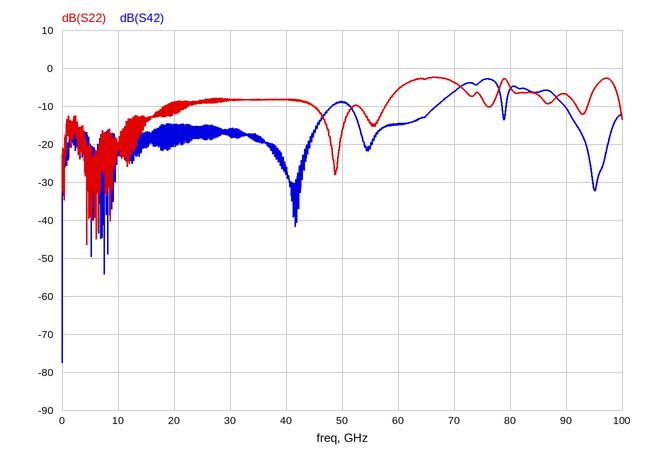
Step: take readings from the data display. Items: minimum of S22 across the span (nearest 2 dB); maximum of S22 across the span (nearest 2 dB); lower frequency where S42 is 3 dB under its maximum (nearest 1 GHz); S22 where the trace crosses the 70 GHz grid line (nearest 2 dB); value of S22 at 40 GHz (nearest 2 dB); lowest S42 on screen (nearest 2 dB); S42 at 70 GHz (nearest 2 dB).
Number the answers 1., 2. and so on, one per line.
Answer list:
1. -46 dB
2. -2 dB
3. 70 GHz
4. -4 dB
5. -8 dB
6. -78 dB
7. -6 dB
